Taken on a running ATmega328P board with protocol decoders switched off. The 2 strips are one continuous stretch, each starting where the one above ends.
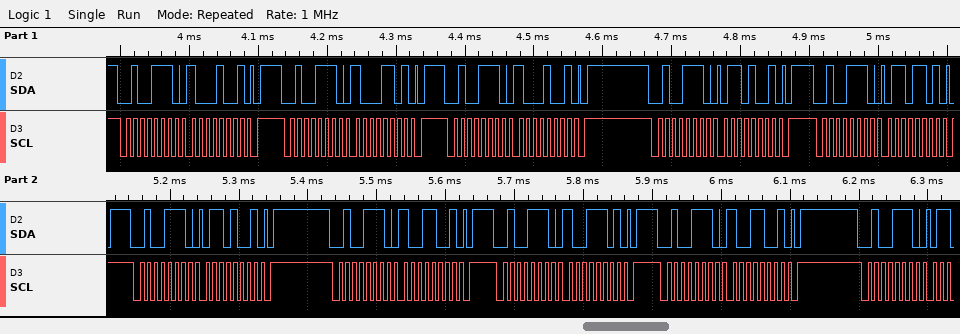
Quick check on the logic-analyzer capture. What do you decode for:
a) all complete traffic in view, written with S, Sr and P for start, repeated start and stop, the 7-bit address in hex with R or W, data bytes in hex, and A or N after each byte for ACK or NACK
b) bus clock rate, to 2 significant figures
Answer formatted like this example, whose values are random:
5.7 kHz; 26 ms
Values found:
S 27W A 89 A P S 27W A 8D A P S 27W A 89 A P S 27W A 69 A P S 27W A 6D A P S 27W A 69 A P S 27W A 99 A P S 27W A 9D A P S 27W A 99 A P S 27W A; 100 kHz
